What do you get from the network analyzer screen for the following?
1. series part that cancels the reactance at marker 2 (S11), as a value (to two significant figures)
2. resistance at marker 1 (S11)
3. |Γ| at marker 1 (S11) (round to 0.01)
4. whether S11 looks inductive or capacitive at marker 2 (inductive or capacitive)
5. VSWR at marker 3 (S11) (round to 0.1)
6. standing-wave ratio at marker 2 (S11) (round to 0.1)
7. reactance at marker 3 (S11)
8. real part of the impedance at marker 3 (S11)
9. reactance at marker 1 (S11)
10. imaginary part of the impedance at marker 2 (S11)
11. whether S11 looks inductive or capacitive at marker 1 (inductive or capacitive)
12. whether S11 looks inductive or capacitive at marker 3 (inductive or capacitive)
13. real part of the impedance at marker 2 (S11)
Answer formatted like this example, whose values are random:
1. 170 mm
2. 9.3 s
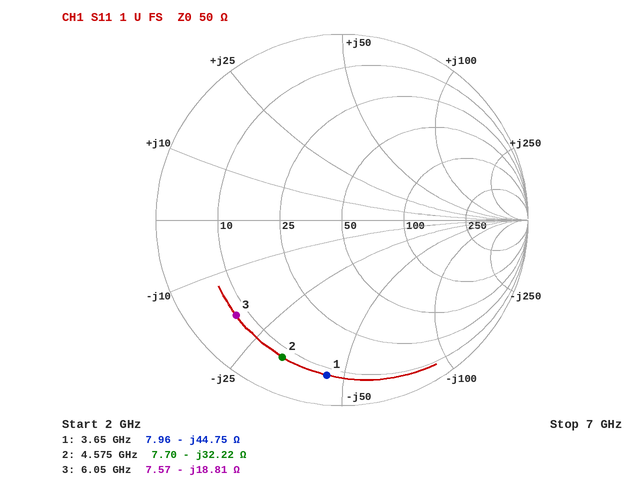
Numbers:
1. 1.1 nH
2. 7.96 Ω
3. 0.84
4. capacitive
5. 7.6
6. 9.2
7. -18.81 Ω
8. 7.57 Ω
9. -44.75 Ω
10. -32.22 Ω
11. capacitive
12. capacitive
13. 7.70 Ω
